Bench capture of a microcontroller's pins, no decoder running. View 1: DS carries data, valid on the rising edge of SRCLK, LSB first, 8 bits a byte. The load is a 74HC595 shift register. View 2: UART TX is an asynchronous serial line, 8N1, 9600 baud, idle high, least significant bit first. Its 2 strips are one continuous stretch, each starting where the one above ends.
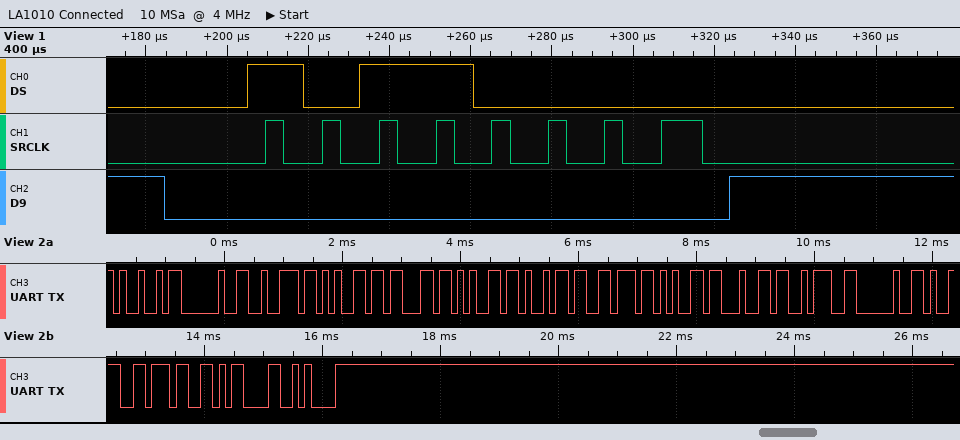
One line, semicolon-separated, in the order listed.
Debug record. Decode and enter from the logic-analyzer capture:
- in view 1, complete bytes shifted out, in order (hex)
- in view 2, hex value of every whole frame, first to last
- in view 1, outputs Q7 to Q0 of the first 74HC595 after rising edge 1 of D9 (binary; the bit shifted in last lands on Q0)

0D; 49 20 72 65 63 65 69 76 65 64 3A 20 39 37 0D 0A; 10110000
